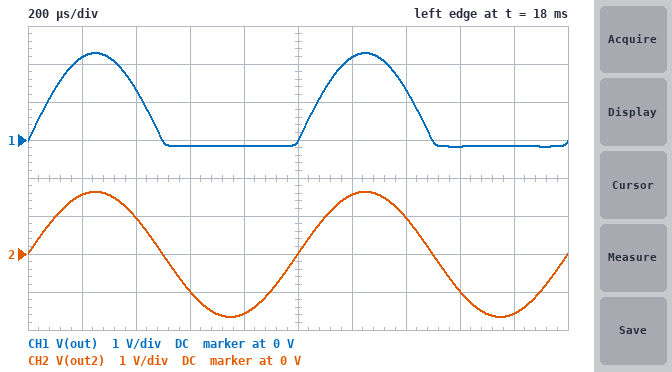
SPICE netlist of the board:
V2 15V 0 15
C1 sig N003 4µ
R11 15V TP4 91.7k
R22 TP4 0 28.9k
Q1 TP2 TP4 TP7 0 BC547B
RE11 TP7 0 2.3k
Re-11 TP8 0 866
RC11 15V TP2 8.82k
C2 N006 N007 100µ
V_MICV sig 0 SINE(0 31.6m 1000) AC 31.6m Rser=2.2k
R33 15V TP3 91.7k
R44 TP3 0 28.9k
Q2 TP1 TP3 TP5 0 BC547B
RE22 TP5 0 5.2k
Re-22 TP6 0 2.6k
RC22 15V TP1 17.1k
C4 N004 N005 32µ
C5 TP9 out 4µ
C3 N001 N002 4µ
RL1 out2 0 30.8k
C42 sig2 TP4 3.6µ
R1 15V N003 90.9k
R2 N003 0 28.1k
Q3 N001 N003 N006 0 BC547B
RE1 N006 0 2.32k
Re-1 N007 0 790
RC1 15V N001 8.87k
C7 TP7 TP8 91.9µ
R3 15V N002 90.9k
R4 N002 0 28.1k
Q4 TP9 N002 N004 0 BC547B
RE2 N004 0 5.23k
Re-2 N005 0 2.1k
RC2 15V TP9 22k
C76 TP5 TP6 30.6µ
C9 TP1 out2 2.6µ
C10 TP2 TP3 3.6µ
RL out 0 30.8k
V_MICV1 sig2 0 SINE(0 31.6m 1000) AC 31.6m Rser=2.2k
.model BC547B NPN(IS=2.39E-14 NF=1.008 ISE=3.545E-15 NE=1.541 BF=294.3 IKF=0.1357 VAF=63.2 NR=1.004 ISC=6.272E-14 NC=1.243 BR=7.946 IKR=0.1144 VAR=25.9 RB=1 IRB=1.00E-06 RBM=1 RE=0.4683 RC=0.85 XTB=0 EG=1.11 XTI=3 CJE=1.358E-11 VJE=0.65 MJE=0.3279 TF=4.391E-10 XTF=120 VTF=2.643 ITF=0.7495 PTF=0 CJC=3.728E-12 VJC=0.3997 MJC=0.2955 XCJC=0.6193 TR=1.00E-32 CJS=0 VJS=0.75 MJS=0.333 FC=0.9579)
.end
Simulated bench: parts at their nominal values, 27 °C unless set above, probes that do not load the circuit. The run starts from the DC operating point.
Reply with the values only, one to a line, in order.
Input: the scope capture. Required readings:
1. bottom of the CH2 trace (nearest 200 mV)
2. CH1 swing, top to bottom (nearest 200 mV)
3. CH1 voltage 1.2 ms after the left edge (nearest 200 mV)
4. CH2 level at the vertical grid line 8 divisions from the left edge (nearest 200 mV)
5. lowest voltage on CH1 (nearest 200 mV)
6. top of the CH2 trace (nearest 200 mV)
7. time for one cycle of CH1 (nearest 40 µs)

-1.6 V
2.4 V
2.2 V
-1.0 V
-200 mV
1.6 V
1.00 ms
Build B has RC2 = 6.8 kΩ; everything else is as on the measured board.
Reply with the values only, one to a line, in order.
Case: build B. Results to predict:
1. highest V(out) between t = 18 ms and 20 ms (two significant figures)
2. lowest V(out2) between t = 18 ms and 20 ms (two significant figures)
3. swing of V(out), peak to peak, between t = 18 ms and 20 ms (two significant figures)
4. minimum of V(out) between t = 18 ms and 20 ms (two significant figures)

1.0 V
-1.7 V
2.0 V
-1.0 V
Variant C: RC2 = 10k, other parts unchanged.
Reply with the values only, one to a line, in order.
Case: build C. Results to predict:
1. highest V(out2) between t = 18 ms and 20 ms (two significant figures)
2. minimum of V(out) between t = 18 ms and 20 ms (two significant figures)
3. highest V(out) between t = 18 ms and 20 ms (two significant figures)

1.6 V
-1.4 V
1.4 V
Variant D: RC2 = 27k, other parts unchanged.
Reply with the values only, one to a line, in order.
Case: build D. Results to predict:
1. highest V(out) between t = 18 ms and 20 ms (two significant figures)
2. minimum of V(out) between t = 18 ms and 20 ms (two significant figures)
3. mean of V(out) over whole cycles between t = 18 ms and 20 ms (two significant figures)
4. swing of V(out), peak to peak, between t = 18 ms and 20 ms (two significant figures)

1.3 V
-49 mV
270 mV
1.4 V
